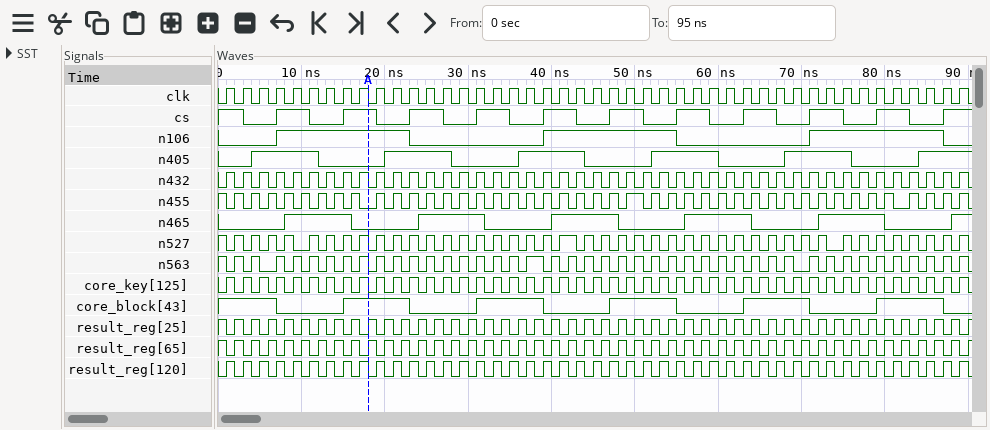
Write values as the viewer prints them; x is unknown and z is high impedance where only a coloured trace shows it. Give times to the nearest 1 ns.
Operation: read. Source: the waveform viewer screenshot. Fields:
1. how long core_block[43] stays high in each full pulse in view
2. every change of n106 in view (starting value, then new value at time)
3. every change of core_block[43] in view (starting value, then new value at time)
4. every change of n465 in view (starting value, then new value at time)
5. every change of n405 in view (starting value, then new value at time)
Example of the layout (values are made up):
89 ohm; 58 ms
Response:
8 ns, 8 ns, 8 ns, 8 ns, 8 ns; 0, 1 at 7 ns, 0 at 23 ns, 1 at 39 ns, 0 at 55 ns, 1 at 71 ns, 0 at 87 ns; 1, 0 at 7 ns, 1 at 15 ns, 0 at 23 ns, 1 at 31 ns, 0 at 39 ns, 1 at 47 ns, 0 at 55 ns, 1 at 63 ns, 0 at 71 ns, 1 at 79 ns, 0 at 87 ns; 0, 1 at 8 ns, 0 at 16 ns, 1 at 24 ns, 0 at 32 ns, 1 at 40 ns, 0 at 48 ns, 1 at 56 ns, 0 at 64 ns, 1 at 72 ns, 0 at 80 ns, 1 at 88 ns; 0, 1 at 4 ns, 0 at 12 ns, 1 at 20 ns, 0 at 28 ns, 1 at 36 ns, 0 at 44 ns, 1 at 52 ns, 0 at 60 ns, 1 at 68 ns, 0 at 76 ns, 1 at 84 ns
